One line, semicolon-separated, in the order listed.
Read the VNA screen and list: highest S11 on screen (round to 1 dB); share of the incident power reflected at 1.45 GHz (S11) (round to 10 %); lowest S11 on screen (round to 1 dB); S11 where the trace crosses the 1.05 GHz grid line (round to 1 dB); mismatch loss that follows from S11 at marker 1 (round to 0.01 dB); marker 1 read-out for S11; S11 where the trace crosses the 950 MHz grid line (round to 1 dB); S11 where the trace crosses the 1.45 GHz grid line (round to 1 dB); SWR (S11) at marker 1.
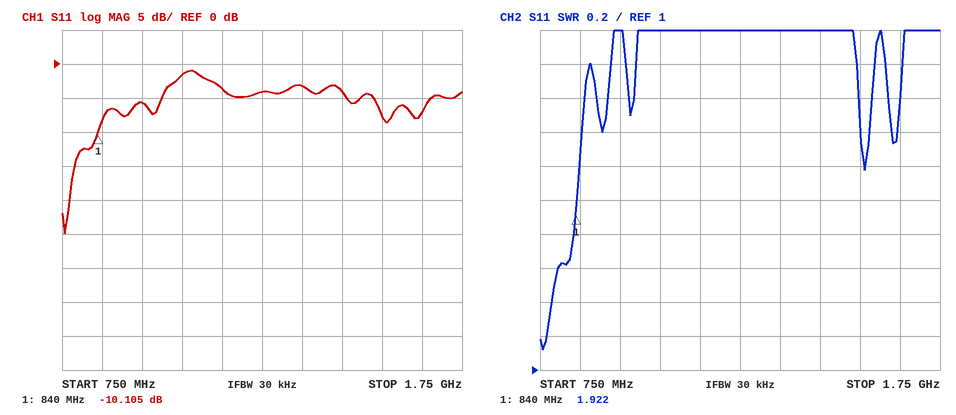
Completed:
-1 dB; 40 %; -25 dB; -2 dB; 0.45 dB; -10.105 dB; -6 dB; -4 dB; 1.922
